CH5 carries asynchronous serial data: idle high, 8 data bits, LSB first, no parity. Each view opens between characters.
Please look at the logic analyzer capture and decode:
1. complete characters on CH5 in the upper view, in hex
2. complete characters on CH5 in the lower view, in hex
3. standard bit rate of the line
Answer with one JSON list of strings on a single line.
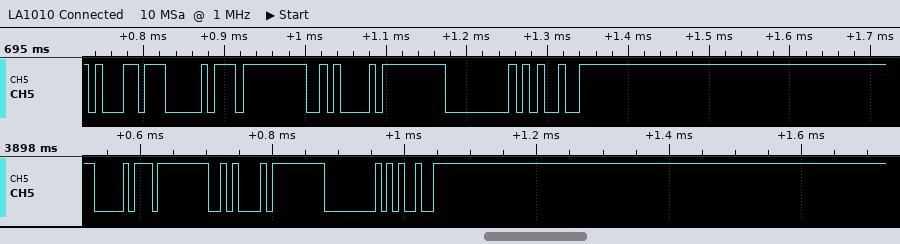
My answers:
["B1, D0, FF, 0A, FF, 00, 25", "D0, FF, 0A, FF, 00, 25", "115200 baud"]
